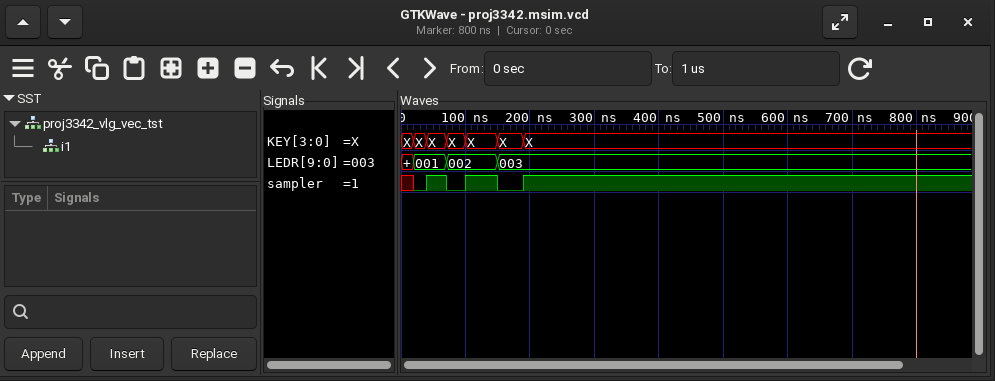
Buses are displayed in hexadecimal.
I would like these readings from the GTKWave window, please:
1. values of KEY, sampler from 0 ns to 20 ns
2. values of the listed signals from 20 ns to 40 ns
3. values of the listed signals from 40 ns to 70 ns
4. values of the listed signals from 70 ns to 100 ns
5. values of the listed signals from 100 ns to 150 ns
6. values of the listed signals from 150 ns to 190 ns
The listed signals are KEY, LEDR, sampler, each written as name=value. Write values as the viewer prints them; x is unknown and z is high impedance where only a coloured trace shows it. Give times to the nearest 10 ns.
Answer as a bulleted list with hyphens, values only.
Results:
- KEY=X, sampler=x
- KEY=X, LEDR=001, sampler=0
- KEY=X, LEDR=001, sampler=1
- KEY=X, LEDR=002, sampler=0
- KEY=X, LEDR=002, sampler=1
- KEY=X, LEDR=003, sampler=0
